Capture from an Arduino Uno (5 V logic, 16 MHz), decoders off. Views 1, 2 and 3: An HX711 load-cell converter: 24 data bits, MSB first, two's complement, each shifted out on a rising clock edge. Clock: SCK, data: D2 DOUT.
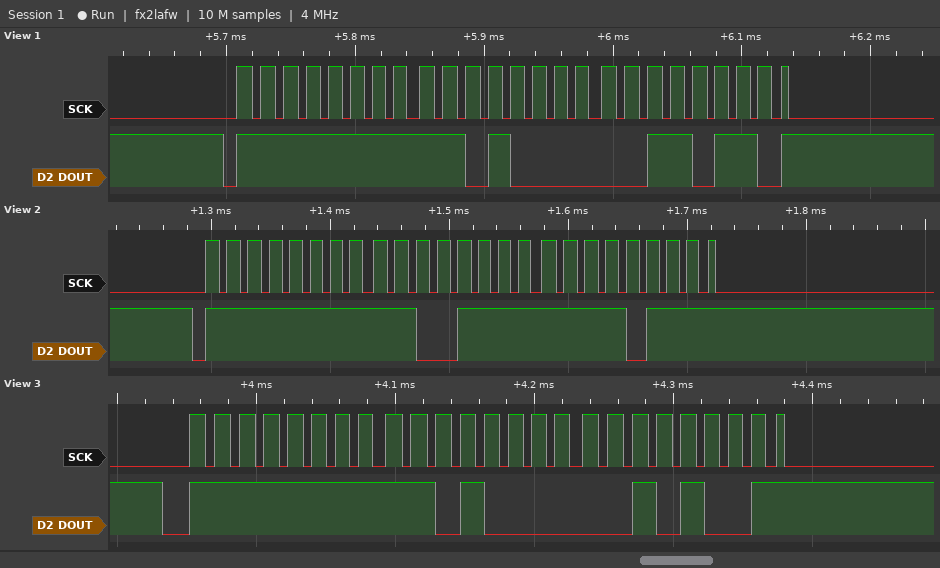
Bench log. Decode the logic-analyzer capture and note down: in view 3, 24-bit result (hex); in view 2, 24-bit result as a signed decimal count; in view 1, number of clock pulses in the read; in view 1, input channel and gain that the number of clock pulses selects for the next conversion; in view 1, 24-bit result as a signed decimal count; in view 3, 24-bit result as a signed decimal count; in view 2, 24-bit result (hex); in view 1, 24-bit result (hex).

0xFFD029
-12297
25
channel A, gain 128
-12234
-12247
0xFFCFF7
0xFFD036
